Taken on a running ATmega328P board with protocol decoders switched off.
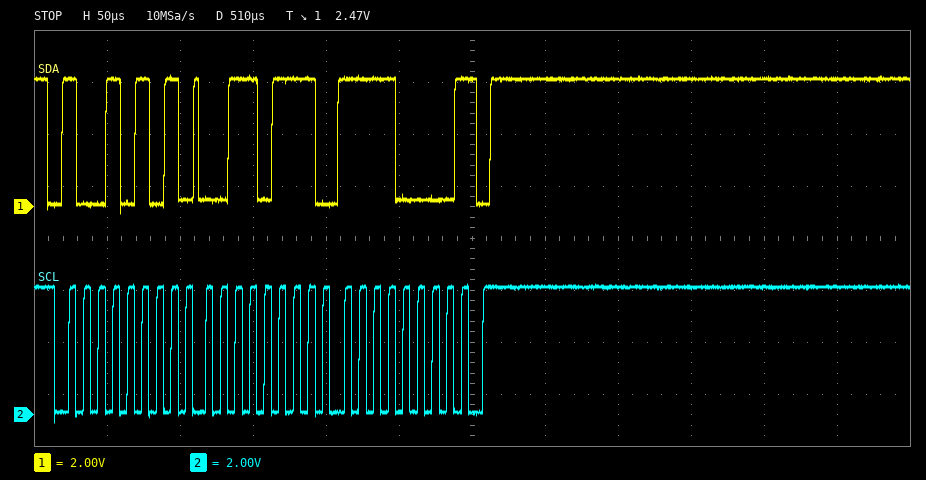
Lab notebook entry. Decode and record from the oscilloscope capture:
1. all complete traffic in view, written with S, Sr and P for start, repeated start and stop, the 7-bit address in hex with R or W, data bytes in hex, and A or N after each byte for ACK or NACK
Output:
S 4AR A 37 A F0 N P
